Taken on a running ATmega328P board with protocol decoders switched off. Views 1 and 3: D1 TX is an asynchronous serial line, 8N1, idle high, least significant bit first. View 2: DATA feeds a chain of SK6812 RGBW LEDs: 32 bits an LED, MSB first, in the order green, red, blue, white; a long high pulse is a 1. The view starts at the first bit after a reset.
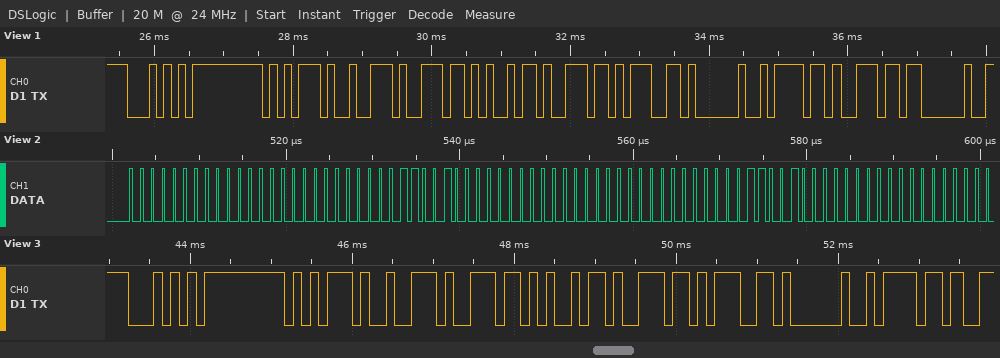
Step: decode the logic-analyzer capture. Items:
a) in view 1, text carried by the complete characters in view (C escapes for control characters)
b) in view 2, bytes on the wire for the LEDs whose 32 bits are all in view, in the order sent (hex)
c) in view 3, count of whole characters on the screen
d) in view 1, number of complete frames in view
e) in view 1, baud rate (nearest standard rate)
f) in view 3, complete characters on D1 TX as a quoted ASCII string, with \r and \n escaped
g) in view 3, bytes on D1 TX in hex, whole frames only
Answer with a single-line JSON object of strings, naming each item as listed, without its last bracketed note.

{"in view 1, text carried by the complete characters in view": "\"Turning on \"", "in view 2, bytes on the wire for the LEDs whose 32 bits are all in view, in the order sent": "00 00 00 64 00 00 00 64", "in view 3, count of whole characters on the screen": "9", "in view 1, number of complete frames in view": "11", "in view 1, baud rate": "9600 baud", "in view 3, complete characters on D1 TX as a quoted ASCII string, with \\r and \\n escaped": "\"Turning o\"", "in view 3, bytes on D1 TX in hex, whole frames only": "54 75 72 6E 69 6E 67 20 6F"}
